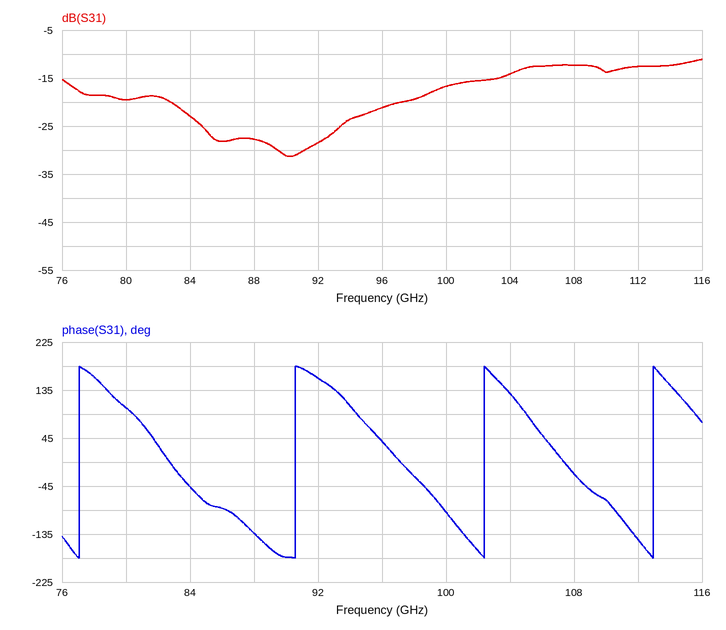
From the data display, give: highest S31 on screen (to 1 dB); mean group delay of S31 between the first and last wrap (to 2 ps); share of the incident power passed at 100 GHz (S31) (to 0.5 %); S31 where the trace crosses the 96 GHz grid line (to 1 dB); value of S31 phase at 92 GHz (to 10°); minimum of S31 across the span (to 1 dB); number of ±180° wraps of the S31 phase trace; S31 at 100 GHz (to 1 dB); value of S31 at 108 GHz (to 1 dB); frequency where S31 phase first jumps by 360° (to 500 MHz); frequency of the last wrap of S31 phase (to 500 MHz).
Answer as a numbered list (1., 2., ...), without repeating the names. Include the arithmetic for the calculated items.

1. -11 dB
2. 3 cycles / (113.0 GHz − 77.0 GHz) ≈ 83.3 ps, so 84 ps to the nearest 2 ps
3. 10^(-17/10) ≈ 2.0 %
4. -21 dB
5. 160°
6. -31 dB
7. 4
8. -17 dB
9. -12 dB
10. 77.0 GHz
11. 113.0 GHz
